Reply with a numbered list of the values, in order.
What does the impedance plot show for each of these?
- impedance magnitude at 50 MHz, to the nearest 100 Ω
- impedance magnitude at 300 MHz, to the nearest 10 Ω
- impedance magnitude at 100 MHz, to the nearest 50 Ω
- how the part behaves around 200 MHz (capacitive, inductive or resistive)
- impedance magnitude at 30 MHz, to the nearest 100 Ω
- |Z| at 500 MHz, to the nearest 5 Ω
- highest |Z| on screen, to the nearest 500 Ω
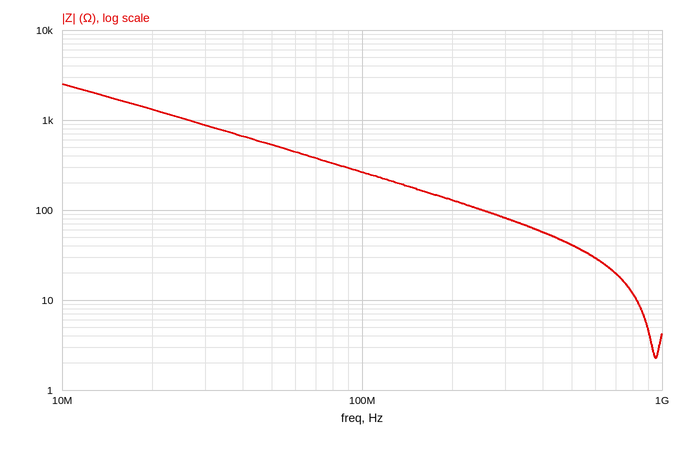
1. 500 Ω
2. 80 Ω
3. 250 Ω
4. capacitive
5. 900 Ω
6. 40 Ω
7. 2.5 kΩ
